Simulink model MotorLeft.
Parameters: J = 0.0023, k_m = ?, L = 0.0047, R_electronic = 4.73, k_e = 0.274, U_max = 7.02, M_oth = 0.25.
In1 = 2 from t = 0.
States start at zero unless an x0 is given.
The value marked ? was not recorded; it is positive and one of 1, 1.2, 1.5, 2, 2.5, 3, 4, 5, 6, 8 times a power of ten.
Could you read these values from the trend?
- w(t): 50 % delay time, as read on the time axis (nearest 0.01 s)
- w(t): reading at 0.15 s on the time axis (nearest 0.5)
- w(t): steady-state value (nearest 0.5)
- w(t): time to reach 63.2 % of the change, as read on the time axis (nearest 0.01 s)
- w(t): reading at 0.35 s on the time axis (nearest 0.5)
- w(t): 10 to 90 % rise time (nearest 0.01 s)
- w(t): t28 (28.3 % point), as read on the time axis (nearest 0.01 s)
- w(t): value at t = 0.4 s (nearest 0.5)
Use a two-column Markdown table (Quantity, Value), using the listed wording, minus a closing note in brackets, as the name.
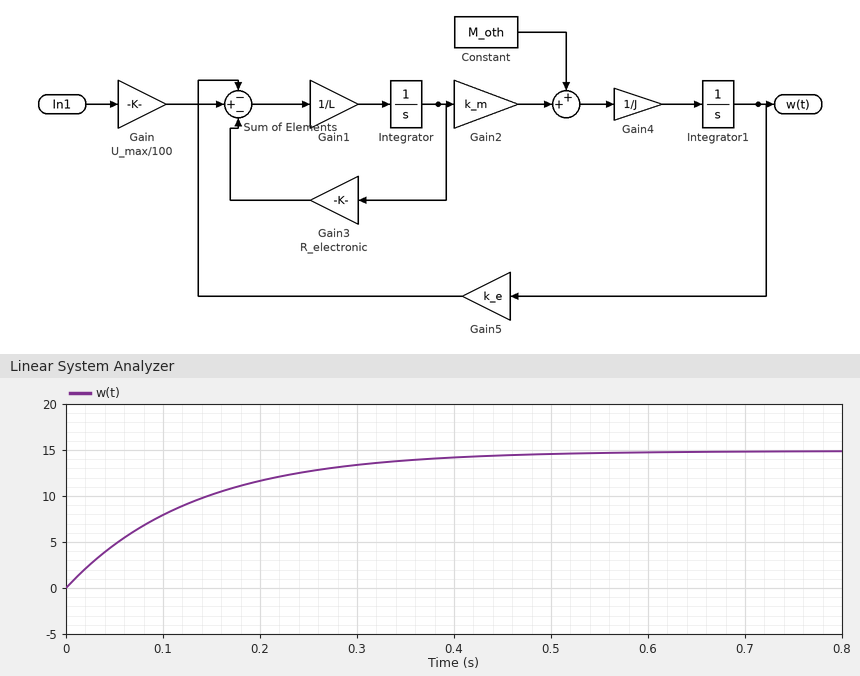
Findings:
| Quantity | Value |
|---|---|
| w(t): 50 % delay time, as read on the time axis | 0.09 s |
| w(t): reading at 0.15 s on the time axis | 10.0 |
| w(t): steady-state value | 15.0 |
| w(t): time to reach 63.2 % of the change, as read on the time axis | 0.13 s |
| w(t): reading at 0.35 s on the time axis | 14.0 |
| w(t): 10 to 90 % rise time | 0.29 s |
| w(t): t28 (28.3 % point), as read on the time axis | 0.04 s |
| w(t): value at t = 0.4 s | 14.0 |
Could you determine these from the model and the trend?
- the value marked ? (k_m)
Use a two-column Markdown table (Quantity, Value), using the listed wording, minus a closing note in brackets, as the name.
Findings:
| Quantity | Value |
|---|---|
| the value marked ? | 0.3 |
